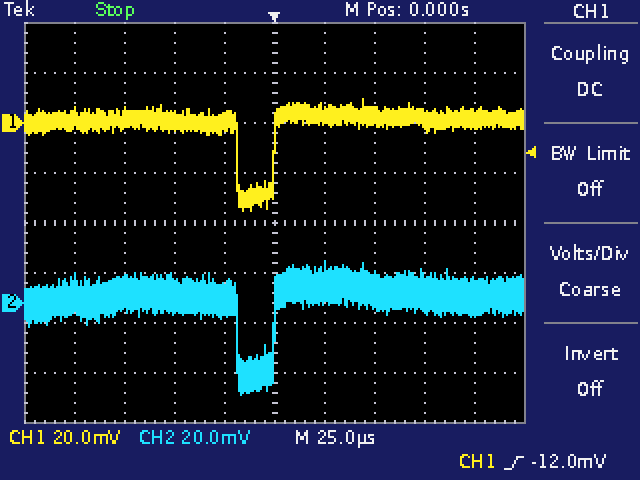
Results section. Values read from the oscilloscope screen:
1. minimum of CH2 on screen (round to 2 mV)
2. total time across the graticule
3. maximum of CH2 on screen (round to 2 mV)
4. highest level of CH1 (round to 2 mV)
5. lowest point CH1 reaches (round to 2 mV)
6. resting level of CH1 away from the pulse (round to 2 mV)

-36 mV
250 µs
16 mV
10 mV
-36 mV
2 mV
